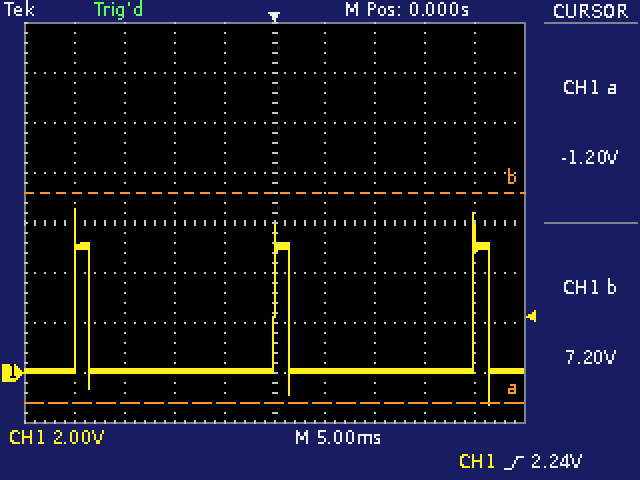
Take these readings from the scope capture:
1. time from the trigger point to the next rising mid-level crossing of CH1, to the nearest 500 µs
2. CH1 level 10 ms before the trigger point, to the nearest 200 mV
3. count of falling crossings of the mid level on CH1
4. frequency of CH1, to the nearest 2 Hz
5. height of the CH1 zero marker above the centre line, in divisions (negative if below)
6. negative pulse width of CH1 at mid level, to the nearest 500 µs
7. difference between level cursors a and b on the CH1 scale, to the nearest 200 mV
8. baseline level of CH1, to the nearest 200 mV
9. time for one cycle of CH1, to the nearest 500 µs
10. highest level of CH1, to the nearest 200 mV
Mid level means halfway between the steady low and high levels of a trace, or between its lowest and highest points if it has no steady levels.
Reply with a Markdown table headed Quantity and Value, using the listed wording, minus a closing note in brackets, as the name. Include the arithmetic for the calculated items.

| Quantity | Value |
|---|---|
| time from the trigger point to the next rising mid-level crossing of CH1, to the nearest 500 µs | 20.0 ms |
| CH1 level 10 ms before the trigger point, to the nearest 200 mV | 0.0 V |
| count of falling crossings of the mid level on CH1 | 3 |
| frequency of CH1, to the nearest 2 Hz | 1 / 20.0 ms ≈ 50 Hz |
| height of the CH1 zero marker above the centre line, in divisions | -3.0 div |
| negative pulse width of CH1 at mid level, to the nearest 500 µs | 18.5 ms |
| difference between level cursors a and b on the CH1 scale, to the nearest 200 mV | 8.4 V |
| baseline level of CH1, to the nearest 200 mV | 0.0 V |
| time for one cycle of CH1, to the nearest 500 µs | 20.0 ms |
| highest level of CH1, to the nearest 200 mV | 6.6 V |
